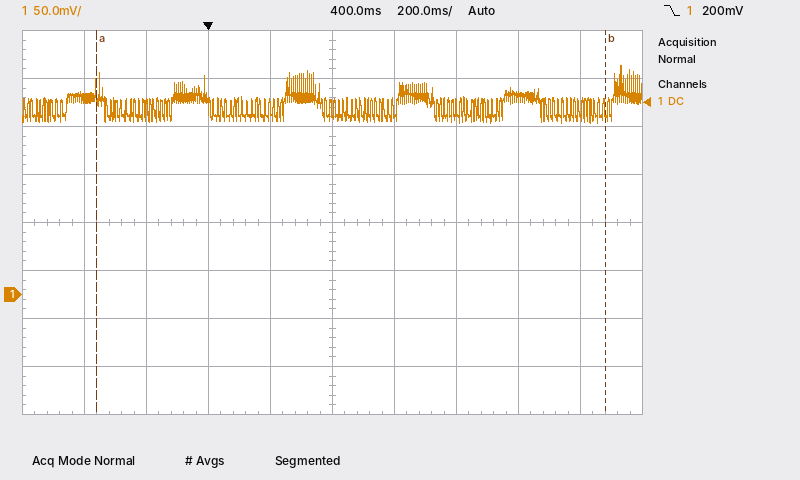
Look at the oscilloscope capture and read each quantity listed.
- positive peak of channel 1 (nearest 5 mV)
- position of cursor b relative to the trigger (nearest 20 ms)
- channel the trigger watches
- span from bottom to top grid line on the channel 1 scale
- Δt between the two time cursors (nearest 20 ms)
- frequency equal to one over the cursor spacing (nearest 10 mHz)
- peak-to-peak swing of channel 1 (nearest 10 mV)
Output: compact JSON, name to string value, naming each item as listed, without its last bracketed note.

{"positive peak of channel 1": "240 mV", "position of cursor b relative to the trigger": "+1.28 s", "channel the trigger watches": "channel 1", "span from bottom to top grid line on the channel 1 scale": "400 mV", "Δt between the two time cursors": "1.64 s", "frequency equal to one over the cursor spacing": "610 mHz", "peak-to-peak swing of channel 1": "60 mV"}
